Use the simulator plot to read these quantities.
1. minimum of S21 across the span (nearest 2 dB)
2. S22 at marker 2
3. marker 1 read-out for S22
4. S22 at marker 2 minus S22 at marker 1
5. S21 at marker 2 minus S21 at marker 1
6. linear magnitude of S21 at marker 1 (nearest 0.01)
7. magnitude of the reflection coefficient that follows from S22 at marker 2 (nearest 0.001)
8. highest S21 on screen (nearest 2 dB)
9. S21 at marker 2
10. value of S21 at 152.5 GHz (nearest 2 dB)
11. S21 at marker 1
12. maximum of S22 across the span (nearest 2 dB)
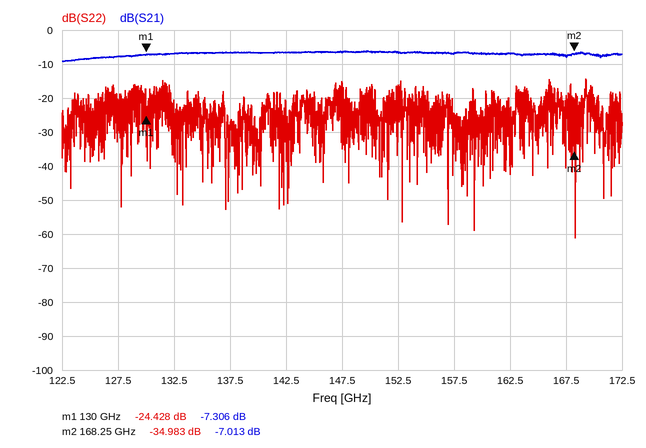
-10 dB
-34.983 dB
-24.428 dB
-10.555 dB
0.293 dB
0.43
0.018
-6 dB
-7.013 dB
-6 dB
-7.306 dB
-14 dB
